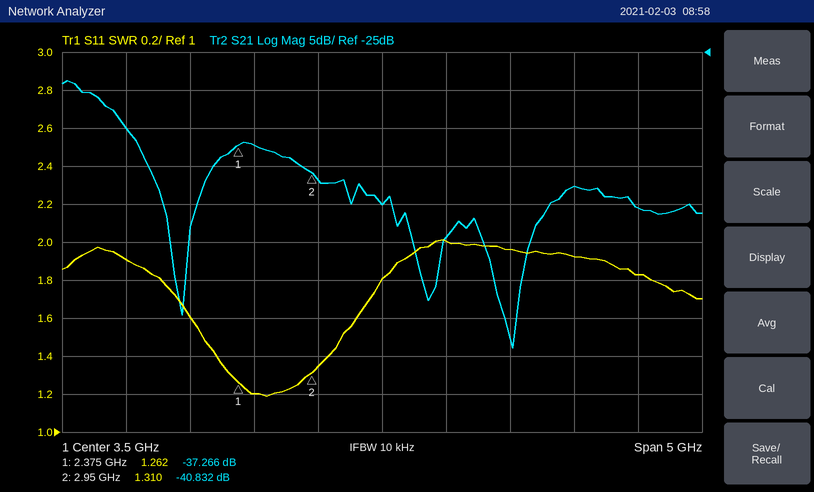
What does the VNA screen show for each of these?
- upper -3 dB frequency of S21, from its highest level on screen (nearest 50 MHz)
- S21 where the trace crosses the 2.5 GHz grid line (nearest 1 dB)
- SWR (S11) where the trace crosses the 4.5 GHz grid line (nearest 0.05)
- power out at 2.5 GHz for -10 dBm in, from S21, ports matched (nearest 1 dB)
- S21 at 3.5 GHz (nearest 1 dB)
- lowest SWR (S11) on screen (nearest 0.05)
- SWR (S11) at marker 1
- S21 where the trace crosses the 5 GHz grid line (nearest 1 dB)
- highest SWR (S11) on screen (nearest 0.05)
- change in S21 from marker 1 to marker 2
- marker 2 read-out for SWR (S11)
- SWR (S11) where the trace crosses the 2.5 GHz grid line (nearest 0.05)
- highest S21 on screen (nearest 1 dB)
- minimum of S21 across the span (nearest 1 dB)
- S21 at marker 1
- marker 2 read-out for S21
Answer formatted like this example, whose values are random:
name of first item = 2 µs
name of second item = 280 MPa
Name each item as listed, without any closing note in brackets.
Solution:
upper -3 dB frequency of S21, from its highest level on screen = 1.30 GHz
S21 where the trace crosses the 2.5 GHz grid line = -37 dB
SWR (S11) where the trace crosses the 4.5 GHz grid line = 1.95
power out at 2.5 GHz for -10 dBm in, from S21, ports matched = -47 dBm
S21 at 3.5 GHz = -45 dB
lowest SWR (S11) on screen = 1.20
SWR (S11) at marker 1 = 1.262
S21 where the trace crosses the 5 GHz grid line = -43 dB
highest SWR (S11) on screen = 2.00
change in S21 from marker 1 to marker 2 = -3.566 dB
marker 2 read-out for SWR = 1.310
SWR (S11) where the trace crosses the 2.5 GHz grid line = 1.20
highest S21 on screen = -29 dB
minimum of S21 across the span = -64 dB
S21 at marker 1 = -37.266 dB
marker 2 read-out for S21 = -40.832 dB
